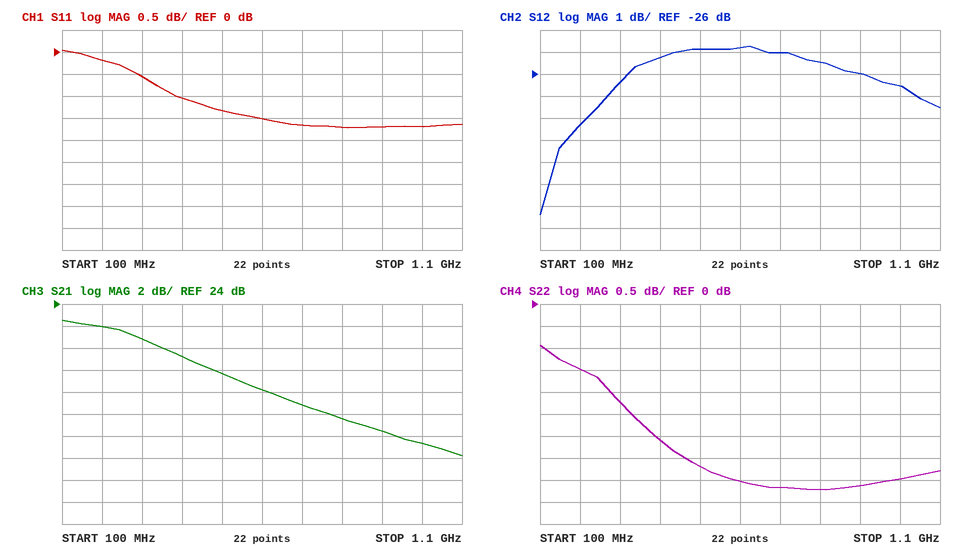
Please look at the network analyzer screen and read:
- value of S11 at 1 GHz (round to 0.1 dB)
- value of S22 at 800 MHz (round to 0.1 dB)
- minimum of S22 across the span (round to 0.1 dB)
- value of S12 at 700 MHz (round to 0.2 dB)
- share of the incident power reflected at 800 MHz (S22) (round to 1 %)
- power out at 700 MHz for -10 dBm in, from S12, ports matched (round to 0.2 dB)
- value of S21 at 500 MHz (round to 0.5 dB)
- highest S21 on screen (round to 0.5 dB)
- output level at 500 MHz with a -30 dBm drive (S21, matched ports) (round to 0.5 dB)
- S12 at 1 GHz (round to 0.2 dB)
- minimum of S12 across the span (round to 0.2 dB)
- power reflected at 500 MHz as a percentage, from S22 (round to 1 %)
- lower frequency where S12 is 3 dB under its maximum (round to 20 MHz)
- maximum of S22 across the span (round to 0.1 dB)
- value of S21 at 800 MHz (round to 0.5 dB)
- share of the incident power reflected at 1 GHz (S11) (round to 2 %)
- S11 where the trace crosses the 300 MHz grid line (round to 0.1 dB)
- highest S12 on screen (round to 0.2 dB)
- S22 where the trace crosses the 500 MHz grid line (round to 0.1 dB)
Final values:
-1.7 dB
-4.2 dB
-4.2 dB
-25.0 dB
38 %
-35.0 dBm
17.5 dB
22.5 dB
-12.5 dBm
-26.6 dB
-32.4 dB
43 %
240 MHz
-0.9 dB
13.5 dB
68 %
-0.6 dB
-24.8 dB
-3.7 dB
